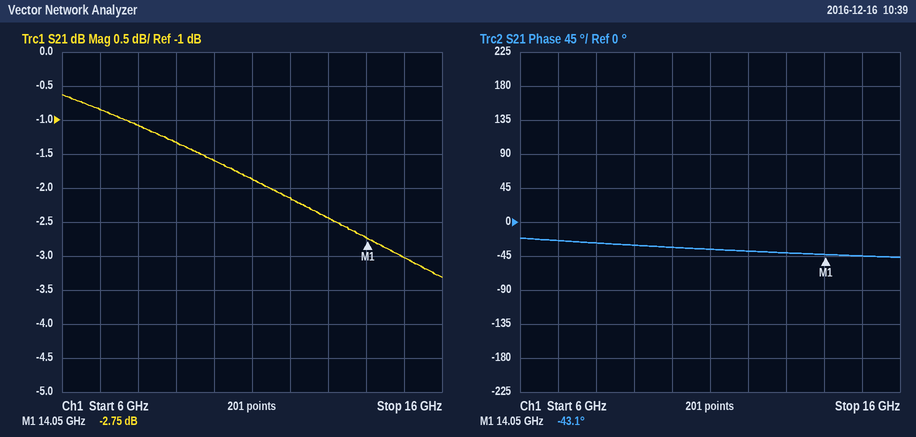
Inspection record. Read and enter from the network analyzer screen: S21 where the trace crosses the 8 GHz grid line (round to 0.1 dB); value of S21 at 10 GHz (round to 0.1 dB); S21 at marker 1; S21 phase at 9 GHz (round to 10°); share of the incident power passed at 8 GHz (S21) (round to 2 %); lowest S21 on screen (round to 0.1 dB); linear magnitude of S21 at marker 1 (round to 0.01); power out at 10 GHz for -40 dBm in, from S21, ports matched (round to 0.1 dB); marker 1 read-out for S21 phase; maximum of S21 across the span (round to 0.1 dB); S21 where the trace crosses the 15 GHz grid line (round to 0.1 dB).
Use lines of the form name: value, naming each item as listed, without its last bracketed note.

S21 where the trace crosses the 8 GHz grid line: -1.1 dB
value of S21 at 10 GHz: -1.6 dB
S21 at marker 1: -2.75 dB
S21 phase at 9 GHz: -30°
share of the incident power passed at 8 GHz (S21): 78 %
lowest S21 on screen: -3.3 dB
linear magnitude of S21 at marker 1: 0.73
power out at 10 GHz for -40 dBm in, from S21, ports matched: -41.6 dBm
marker 1 read-out for S21 phase: -43.1°
maximum of S21 across the span: -0.6 dB
S21 where the trace crosses the 15 GHz grid line: -3.0 dB
